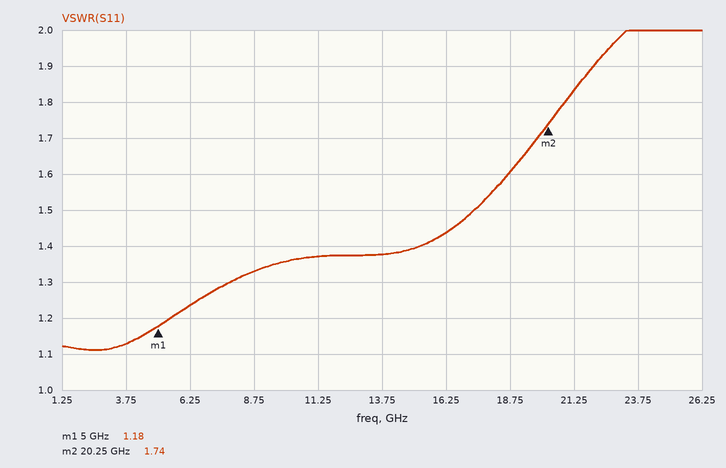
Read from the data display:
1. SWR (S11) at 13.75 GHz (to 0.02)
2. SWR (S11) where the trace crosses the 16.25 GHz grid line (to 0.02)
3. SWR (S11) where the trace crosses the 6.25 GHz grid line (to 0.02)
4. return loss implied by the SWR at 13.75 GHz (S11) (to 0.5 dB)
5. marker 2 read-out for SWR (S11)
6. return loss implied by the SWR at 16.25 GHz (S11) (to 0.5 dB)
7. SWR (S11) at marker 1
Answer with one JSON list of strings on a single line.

["1.38", "1.44", "1.24", "16.0 dB", "1.74", "15.0 dB", "1.18"]
